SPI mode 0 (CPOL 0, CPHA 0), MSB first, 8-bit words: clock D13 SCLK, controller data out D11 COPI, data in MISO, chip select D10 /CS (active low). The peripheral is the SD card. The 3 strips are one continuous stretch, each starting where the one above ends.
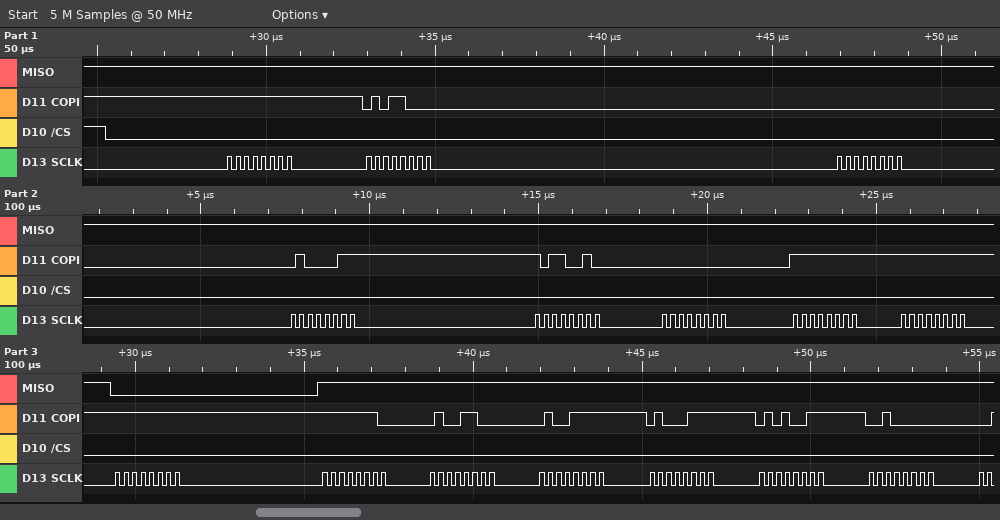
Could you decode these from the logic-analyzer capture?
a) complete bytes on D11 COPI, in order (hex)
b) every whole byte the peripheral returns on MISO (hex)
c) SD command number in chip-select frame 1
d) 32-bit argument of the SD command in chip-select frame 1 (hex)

FF 58 00 43 B2 00 FF FF FF FE 4C 4F 47 53 20
FF FF FF FF FF FF FF FF 00 FF FF FF FF FF FF
CMD24
0x0043B200
